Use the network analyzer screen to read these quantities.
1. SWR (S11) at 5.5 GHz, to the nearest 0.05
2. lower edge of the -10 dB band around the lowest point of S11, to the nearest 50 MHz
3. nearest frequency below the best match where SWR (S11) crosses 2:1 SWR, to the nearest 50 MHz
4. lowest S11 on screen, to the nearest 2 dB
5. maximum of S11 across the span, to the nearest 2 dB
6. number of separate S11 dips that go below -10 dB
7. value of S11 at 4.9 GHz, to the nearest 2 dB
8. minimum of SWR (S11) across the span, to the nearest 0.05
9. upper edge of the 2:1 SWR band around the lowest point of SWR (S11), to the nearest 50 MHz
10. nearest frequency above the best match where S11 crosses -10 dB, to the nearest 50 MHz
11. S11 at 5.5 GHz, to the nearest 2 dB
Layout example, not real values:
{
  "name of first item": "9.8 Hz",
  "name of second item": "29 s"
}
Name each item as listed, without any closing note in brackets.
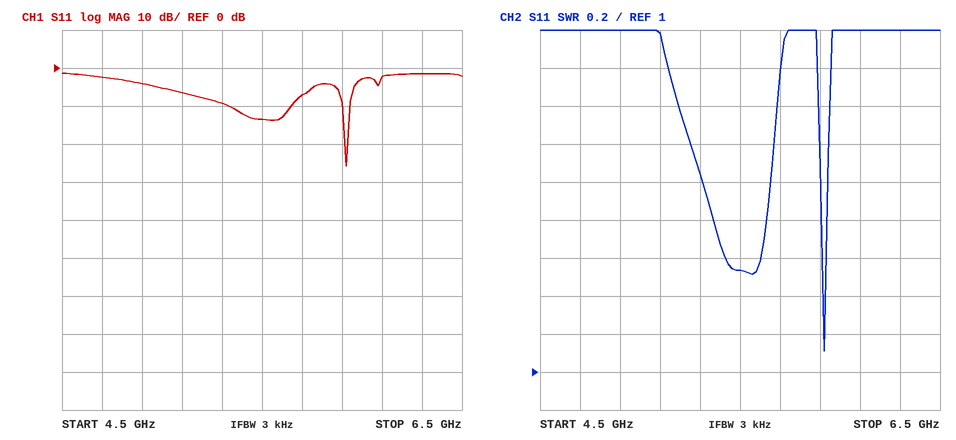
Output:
{
  "SWR (S11) at 5.5 GHz, to the nearest 0.05": "1.55",
  "lower edge of the -10 dB band around the lowest point of S11, to the nearest 50 MHz": "5.90 GHz",
  "nearest frequency below the best match where SWR (S11) crosses 2:1 SWR, to the nearest 50 MHz": "5.90 GHz",
  "lowest S11 on screen, to the nearest 2 dB": "-26 dB",
  "maximum of S11 across the span, to the nearest 2 dB": "-2 dB",
  "number of separate S11 dips that go below -10 dB": "2",
  "value of S11 at 4.9 GHz, to the nearest 2 dB": "-4 dB",
  "minimum of SWR (S11) across the span, to the nearest 0.05": "1.10",
  "upper edge of the 2:1 SWR band around the lowest point of SWR (S11), to the nearest 50 MHz": "5.95 GHz",
  "nearest frequency above the best match where S11 crosses -10 dB, to the nearest 50 MHz": "5.95 GHz",
  "S11 at 5.5 GHz, to the nearest 2 dB": "-14 dB"
}
